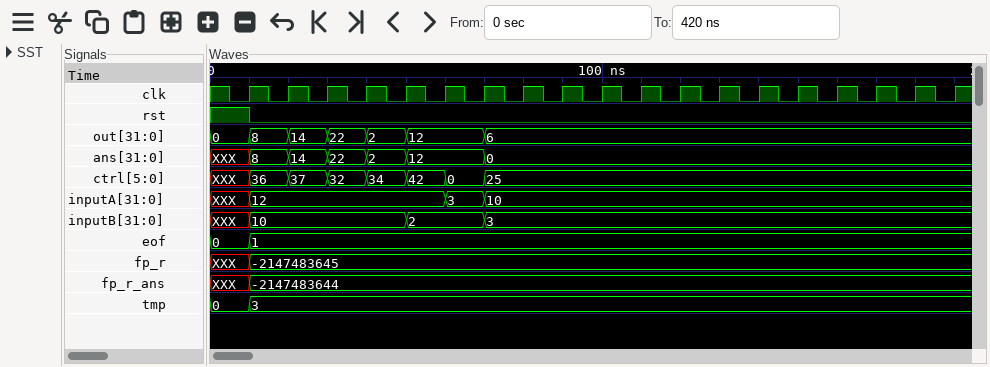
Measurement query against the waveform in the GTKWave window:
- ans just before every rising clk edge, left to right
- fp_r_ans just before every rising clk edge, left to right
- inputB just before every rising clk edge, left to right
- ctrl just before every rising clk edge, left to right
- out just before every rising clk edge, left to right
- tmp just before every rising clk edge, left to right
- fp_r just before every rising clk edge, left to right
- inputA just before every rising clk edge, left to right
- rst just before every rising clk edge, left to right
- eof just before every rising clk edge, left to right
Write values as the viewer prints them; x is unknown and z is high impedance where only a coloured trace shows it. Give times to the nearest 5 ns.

XXX, 8, 14, 22, 2, 12, 12, 0, 0, 0, 0, 0, 0, 0, 0, 0, 0, 0, 0
XXX, -2147483644, -2147483644, -2147483644, -2147483644, -2147483644, -2147483644, -2147483644, -2147483644, -2147483644, -2147483644, -2147483644, -2147483644, -2147483644, -2147483644, -2147483644, -2147483644, -2147483644, -2147483644
XXX, 10, 10, 10, 10, 2, 2, 3, 3, 3, 3, 3, 3, 3, 3, 3, 3, 3, 3
XXX, 36, 37, 32, 34, 42, 0, 25, 25, 25, 25, 25, 25, 25, 25, 25, 25, 25, 25
0, 8, 14, 22, 2, 12, 12, 6, 6, 6, 6, 6, 6, 6, 6, 6, 6, 6, 6
0, 3, 3, 3, 3, 3, 3, 3, 3, 3, 3, 3, 3, 3, 3, 3, 3, 3, 3
XXX, -2147483645, -2147483645, -2147483645, -2147483645, -2147483645, -2147483645, -2147483645, -2147483645, -2147483645, -2147483645, -2147483645, -2147483645, -2147483645, -2147483645, -2147483645, -2147483645, -2147483645, -2147483645
XXX, 12, 12, 12, 12, 12, 3, 10, 10, 10, 10, 10, 10, 10, 10, 10, 10, 10, 10
1 0 0 0 0 0 0 0 0 0 0 0 0 0 0 0 0 0 0
0, 1, 1, 1, 1, 1, 1, 1, 1, 1, 1, 1, 1, 1, 1, 1, 1, 1, 1
